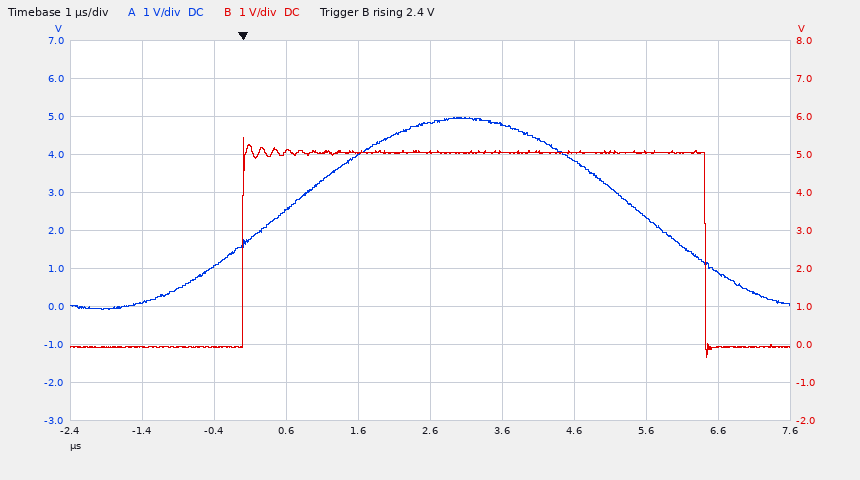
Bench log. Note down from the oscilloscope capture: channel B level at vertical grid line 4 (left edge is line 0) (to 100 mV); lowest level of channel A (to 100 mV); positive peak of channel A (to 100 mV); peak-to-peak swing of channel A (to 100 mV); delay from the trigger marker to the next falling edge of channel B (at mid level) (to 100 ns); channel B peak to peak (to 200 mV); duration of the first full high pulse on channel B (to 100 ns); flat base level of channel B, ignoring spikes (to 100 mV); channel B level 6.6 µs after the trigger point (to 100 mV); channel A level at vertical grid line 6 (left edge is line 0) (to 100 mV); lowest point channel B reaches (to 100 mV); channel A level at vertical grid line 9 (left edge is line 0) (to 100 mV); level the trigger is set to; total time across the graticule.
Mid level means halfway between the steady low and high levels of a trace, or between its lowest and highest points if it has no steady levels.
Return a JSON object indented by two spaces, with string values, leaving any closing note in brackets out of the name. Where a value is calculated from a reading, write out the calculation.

{
  "channel B level at vertical grid line 4 (left edge is line 0)": "5.0 V",
  "lowest level of channel A": "-100 mV",
  "positive peak of channel A": "5.0 V",
  "peak-to-peak swing of channel A": "5.0 V − (-100 mV) = 5.1 V",
  "delay from the trigger marker to the next falling edge of channel B (at mid level)": "6.4 µs",
  "channel B peak to peak": "5.8 V",
  "duration of the first full high pulse on channel B": "6.4 µs",
  "flat base level of channel B, ignoring spikes": "-100 mV",
  "channel B level 6.6 µs after the trigger point": "-100 mV",
  "channel A level at vertical grid line 6 (left edge is line 0)": "4.8 V",
  "lowest point channel B reaches": "-300 mV",
  "channel A level at vertical grid line 9 (left edge is line 0)": "900 mV",
  "level the trigger is set to": "2.4 V",
  "total time across the graticule": "10 µs"
}
